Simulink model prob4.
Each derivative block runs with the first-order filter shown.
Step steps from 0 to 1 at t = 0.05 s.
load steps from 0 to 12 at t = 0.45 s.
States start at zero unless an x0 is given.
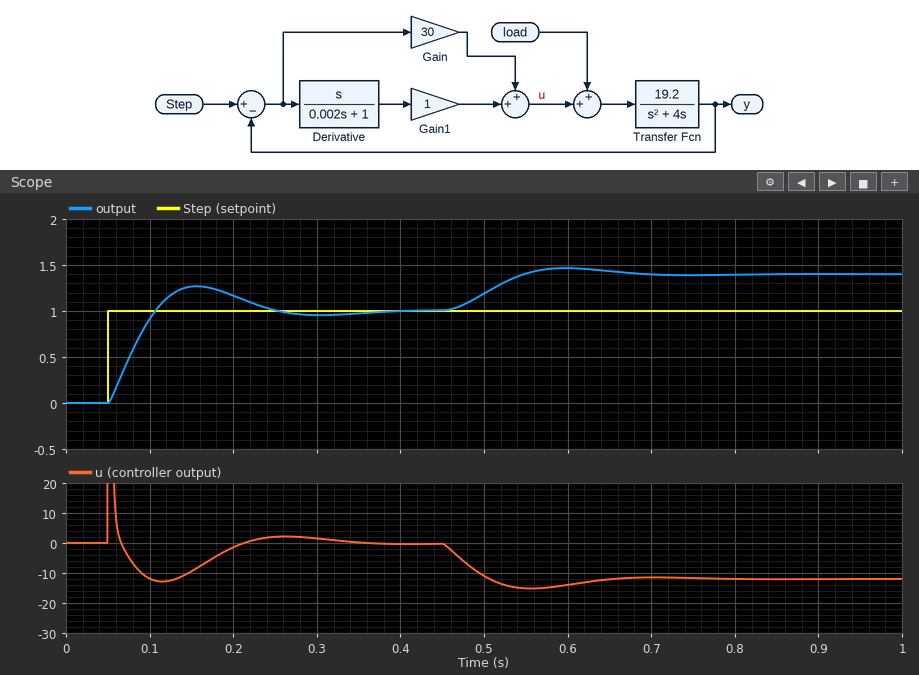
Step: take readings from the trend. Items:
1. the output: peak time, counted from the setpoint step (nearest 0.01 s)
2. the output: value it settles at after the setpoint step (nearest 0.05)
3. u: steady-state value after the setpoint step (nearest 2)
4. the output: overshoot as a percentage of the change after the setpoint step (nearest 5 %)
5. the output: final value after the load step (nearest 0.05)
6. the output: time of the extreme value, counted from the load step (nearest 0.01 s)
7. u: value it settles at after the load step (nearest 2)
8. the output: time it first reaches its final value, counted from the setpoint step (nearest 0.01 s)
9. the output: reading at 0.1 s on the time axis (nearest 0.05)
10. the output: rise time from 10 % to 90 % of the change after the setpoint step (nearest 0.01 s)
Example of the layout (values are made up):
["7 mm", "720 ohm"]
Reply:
["0.11 s", "1.00", "0", "25 %", "1.40", "0.15 s", "-12", "0.06 s", "0.90", "0.04 s"]
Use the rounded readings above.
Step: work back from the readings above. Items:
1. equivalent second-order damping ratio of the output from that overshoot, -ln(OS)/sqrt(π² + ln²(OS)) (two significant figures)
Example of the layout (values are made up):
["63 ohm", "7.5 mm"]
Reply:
["0.40"]
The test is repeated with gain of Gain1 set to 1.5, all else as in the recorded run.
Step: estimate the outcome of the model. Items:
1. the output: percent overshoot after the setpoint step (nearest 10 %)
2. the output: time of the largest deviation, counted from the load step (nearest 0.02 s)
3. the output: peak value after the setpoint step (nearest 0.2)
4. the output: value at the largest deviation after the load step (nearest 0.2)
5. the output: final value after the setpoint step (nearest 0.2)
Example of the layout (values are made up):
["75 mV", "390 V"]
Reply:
["20 %", "0.18 s", "1.2", "1.4", "1.0"]
